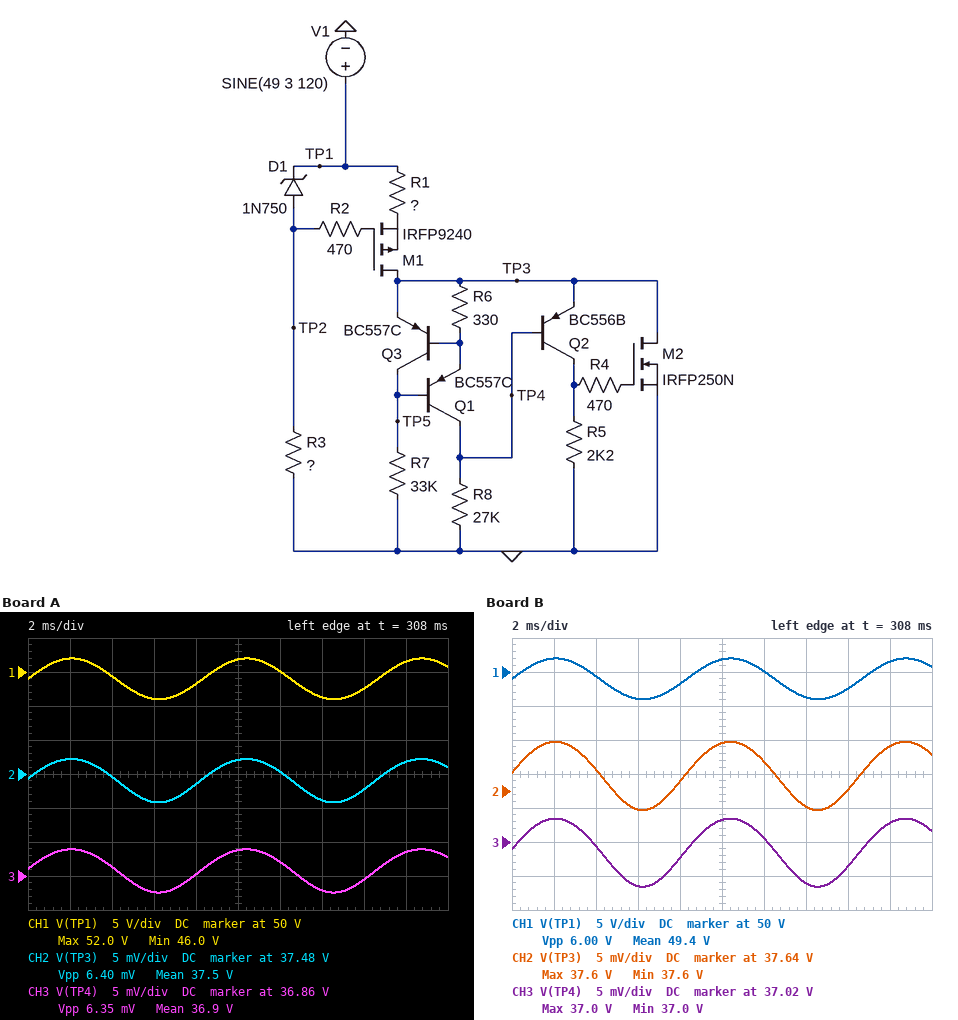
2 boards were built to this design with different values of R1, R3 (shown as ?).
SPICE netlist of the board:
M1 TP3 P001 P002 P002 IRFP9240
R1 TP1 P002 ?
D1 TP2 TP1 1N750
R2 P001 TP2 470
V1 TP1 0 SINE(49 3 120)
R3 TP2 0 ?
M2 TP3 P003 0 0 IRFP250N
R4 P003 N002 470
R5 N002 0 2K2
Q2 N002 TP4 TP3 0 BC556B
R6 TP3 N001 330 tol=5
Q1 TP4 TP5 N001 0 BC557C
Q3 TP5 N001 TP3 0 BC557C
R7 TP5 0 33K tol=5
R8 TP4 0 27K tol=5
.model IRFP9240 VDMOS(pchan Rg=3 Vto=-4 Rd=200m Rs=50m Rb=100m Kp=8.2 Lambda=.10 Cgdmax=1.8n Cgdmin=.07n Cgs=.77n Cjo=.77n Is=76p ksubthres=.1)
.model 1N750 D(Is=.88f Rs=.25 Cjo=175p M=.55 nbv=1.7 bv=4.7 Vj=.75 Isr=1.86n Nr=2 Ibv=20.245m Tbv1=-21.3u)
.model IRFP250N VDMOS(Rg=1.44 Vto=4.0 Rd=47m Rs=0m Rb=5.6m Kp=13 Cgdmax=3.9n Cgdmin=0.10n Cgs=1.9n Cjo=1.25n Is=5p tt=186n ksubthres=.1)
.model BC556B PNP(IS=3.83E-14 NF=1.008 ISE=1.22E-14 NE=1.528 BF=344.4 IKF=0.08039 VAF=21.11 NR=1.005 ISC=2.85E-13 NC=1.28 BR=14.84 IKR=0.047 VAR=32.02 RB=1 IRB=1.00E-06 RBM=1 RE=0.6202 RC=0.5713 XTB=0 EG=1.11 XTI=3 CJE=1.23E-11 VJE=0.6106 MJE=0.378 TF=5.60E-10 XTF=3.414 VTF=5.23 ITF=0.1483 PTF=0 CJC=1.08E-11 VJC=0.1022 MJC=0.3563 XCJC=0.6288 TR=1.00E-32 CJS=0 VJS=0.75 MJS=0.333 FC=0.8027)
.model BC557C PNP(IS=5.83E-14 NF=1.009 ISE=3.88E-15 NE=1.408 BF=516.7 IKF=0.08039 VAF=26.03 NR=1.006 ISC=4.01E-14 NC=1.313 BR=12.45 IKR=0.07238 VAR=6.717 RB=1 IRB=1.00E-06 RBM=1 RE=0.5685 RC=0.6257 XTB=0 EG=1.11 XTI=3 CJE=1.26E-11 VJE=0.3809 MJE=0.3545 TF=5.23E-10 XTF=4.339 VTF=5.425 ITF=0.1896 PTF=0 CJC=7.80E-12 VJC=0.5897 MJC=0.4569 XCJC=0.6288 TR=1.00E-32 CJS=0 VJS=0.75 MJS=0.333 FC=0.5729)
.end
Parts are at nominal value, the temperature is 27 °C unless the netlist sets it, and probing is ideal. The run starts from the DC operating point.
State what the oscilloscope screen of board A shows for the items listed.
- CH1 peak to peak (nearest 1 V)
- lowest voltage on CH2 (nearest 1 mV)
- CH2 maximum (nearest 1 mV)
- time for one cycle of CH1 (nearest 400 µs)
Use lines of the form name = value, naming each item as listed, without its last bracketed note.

CH1 peak to peak = 6 V
lowest voltage on CH2 = 37.471 V
CH2 maximum = 37.477 V
time for one cycle of CH1 = 8.4 ms
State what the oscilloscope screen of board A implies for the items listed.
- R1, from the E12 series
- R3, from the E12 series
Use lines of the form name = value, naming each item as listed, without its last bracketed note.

R1, from the E12 series = 12 Ω
R3, from the E12 series = 5.6 kΩ
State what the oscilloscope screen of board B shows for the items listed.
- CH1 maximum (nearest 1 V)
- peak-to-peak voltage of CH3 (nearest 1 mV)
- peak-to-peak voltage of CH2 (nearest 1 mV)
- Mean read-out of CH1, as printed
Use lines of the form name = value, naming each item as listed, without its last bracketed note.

CH1 maximum = 52 V
peak-to-peak voltage of CH3 = 10 mV
peak-to-peak voltage of CH2 = 10 mV
Mean read-out of CH1, as printed = 49.4 V
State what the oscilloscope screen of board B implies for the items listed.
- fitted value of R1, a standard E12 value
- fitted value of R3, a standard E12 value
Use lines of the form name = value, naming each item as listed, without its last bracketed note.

fitted value of R1, a standard E12 value = 3.9 Ω
fitted value of R3, a standard E12 value = 12 kΩ
